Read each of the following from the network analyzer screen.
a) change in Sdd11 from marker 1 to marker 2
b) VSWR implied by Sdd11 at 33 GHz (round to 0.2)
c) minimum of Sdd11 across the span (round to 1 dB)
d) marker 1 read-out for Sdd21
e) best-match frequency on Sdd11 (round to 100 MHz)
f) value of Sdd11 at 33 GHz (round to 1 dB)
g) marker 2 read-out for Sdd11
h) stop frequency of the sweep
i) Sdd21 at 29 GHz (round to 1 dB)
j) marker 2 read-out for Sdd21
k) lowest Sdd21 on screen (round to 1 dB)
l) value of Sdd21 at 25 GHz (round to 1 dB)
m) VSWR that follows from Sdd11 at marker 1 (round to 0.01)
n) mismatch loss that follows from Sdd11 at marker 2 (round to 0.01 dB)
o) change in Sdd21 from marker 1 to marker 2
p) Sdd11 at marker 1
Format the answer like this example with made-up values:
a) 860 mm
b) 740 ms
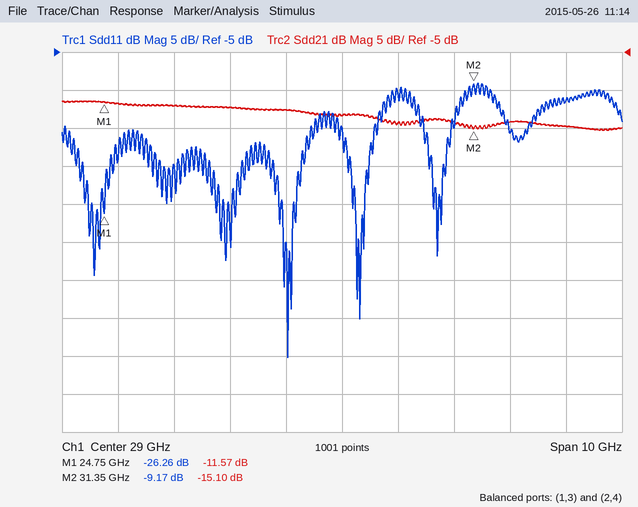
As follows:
a) 17.09 dB
b) 1.8
c) -45 dB
d) -11.57 dB
e) 28.0 GHz
f) -11 dB
g) -9.17 dB
h) 34 GHz
i) -13 dB
j) -15.10 dB
k) -15 dB
l) -12 dB
m) 1.10
n) 0.56 dB
o) -3.53 dB
p) -26.26 dB
